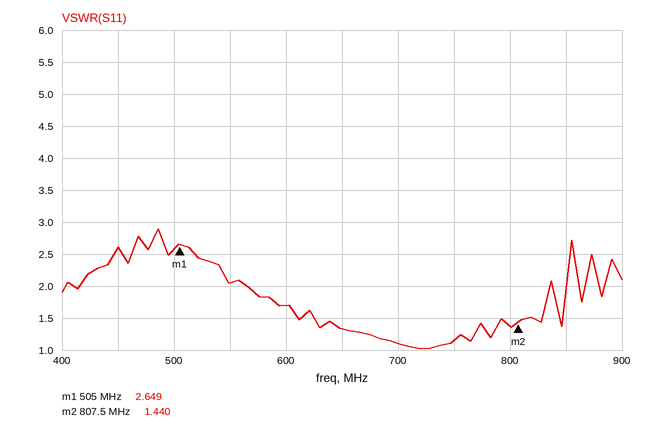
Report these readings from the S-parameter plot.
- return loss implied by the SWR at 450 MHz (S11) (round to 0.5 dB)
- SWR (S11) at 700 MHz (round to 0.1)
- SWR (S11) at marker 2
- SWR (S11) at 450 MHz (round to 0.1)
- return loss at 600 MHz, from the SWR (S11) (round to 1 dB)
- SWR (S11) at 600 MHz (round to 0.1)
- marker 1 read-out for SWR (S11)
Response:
7.0 dB
1.1
1.440
2.6
12 dB
1.7
2.649
